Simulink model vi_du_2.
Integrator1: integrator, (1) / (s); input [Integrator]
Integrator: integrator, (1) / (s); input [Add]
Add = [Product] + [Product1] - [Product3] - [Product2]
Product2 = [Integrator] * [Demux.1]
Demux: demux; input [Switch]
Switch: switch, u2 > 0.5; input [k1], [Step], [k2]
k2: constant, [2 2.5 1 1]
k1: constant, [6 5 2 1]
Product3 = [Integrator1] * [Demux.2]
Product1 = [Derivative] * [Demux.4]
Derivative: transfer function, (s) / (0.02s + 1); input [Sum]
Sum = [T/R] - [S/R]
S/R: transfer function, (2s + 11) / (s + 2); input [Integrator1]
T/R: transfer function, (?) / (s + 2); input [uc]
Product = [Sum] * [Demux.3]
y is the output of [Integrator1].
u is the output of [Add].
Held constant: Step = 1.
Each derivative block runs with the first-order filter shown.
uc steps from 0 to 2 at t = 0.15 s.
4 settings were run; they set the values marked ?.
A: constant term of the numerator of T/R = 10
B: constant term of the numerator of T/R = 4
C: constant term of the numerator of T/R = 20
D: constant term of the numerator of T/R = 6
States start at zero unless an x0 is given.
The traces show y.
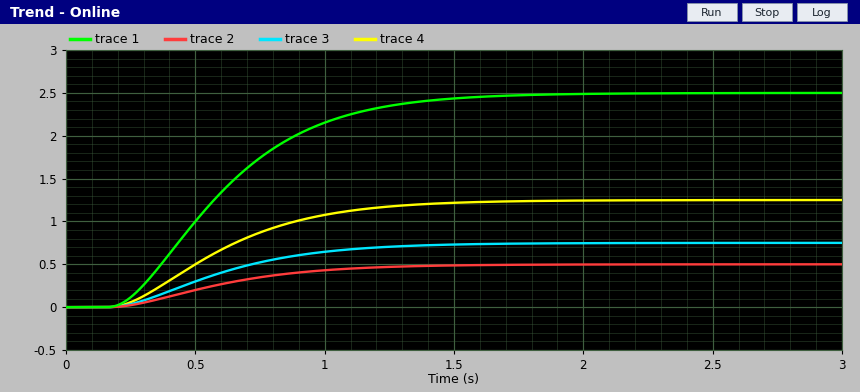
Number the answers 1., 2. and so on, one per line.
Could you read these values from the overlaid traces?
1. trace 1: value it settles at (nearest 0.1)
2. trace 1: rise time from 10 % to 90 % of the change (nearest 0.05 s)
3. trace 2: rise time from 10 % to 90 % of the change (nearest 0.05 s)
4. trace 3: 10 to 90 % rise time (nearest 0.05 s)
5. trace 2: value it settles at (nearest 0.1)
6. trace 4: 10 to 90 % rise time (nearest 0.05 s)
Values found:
1. 2.5
2. 0.80 s
3. 0.80 s
4. 0.80 s
5. 0.5
6. 0.80 s
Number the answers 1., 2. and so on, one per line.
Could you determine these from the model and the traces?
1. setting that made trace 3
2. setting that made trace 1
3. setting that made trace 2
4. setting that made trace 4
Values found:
1. D
2. C
3. B
4. A
